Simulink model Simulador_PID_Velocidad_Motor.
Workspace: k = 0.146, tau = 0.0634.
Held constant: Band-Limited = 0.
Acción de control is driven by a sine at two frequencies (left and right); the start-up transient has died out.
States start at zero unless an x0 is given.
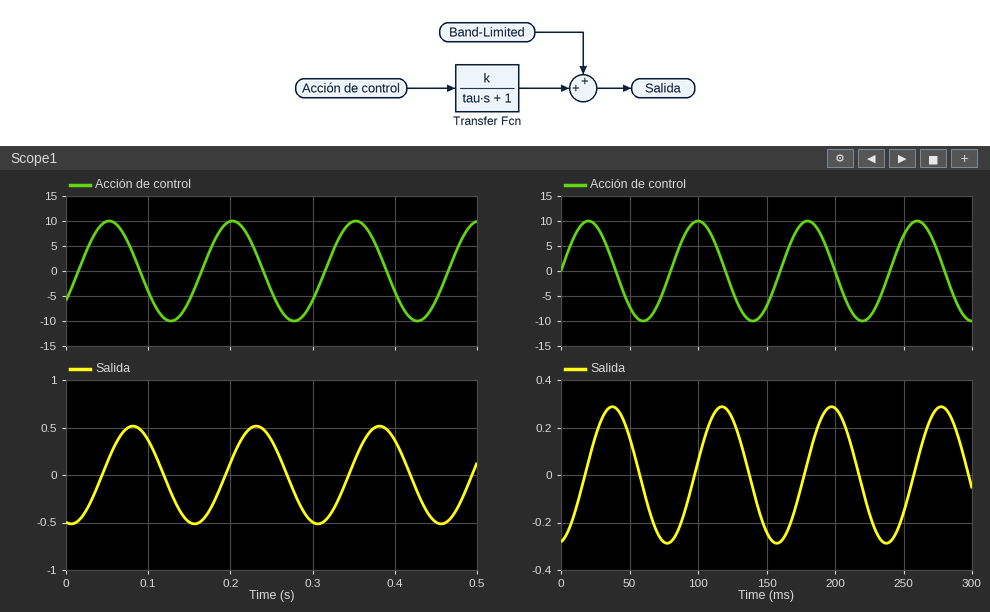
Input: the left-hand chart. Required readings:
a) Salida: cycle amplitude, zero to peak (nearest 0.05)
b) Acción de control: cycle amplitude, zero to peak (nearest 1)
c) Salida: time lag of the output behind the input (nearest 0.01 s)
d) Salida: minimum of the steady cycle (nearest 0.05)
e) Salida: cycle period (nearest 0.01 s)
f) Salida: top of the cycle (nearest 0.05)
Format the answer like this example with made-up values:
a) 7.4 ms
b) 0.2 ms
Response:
a) 0.50
b) 10
c) 0.03 s
d) -0.50
e) 0.15 s
f) 0.50
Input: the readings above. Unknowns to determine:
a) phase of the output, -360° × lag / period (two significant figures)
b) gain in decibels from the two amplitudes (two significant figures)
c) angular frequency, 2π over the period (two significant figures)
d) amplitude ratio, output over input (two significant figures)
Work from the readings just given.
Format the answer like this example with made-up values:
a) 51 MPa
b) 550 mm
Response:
a) -72°
b) -26 dB
c) 42 rad/s
d) 0.050
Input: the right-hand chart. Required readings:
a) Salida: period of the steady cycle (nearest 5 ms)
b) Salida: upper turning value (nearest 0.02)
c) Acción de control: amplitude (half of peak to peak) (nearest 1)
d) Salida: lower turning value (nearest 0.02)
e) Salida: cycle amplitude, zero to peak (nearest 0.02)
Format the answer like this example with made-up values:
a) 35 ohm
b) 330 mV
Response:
a) 80 ms
b) 0.28
c) 10
d) -0.28
e) 0.28
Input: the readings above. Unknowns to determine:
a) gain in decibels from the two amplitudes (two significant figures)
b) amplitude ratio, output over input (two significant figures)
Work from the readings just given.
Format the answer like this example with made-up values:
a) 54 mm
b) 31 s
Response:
a) -31 dB
b) 0.028
